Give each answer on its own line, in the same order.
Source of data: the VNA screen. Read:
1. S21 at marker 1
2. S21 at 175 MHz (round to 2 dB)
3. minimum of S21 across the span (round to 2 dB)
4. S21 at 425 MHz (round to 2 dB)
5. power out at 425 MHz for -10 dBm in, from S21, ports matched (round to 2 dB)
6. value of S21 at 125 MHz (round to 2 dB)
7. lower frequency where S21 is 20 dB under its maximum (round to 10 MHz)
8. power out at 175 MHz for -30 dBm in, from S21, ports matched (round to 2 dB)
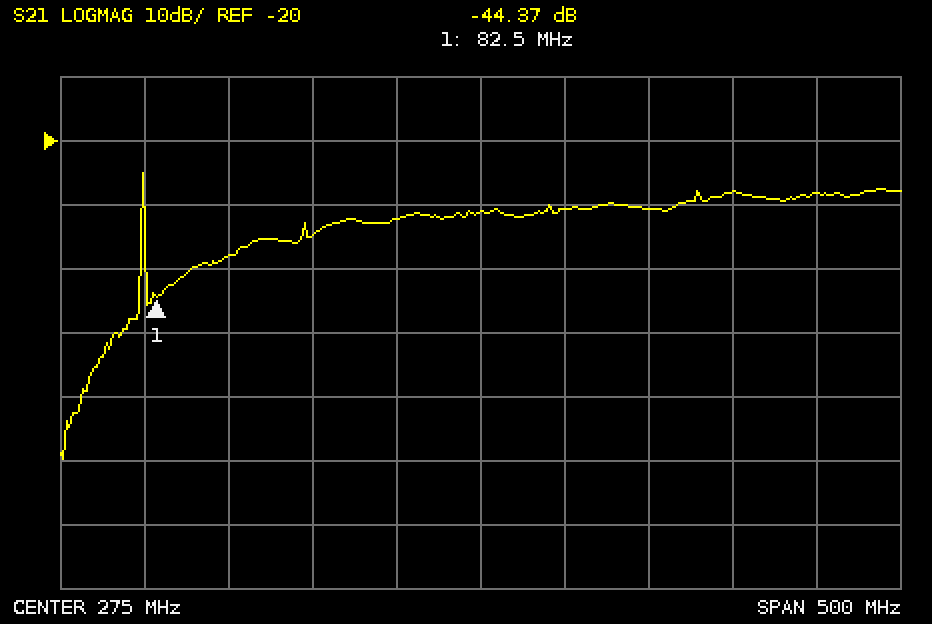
-44.37 dB
-34 dB
-70 dB
-28 dB
-38 dBm
-38 dB
70 MHz
-64 dBm
